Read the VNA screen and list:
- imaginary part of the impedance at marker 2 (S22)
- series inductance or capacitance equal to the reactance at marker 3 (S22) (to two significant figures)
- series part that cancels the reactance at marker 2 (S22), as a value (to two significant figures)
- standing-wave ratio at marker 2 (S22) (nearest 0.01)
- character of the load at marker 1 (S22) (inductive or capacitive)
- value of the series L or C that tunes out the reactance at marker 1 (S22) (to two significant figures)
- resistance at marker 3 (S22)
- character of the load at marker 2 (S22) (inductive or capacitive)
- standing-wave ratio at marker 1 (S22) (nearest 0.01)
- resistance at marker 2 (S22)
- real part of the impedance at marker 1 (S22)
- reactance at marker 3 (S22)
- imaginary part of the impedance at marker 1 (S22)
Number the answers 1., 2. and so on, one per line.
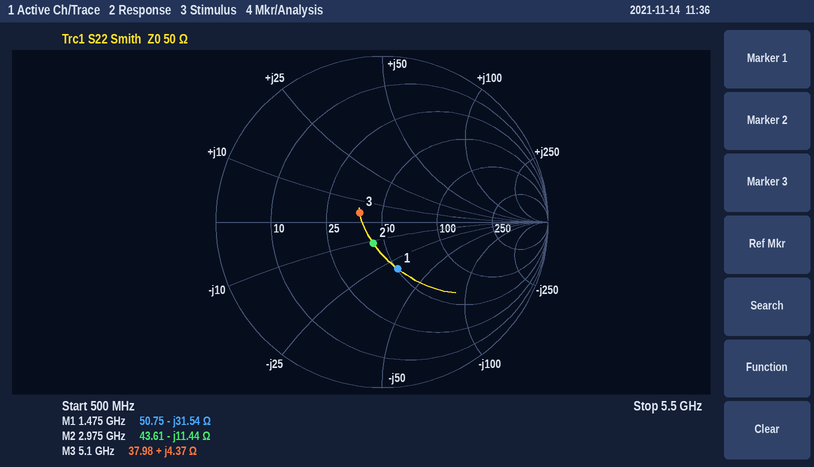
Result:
1. -11.44 Ω
2. 140 pH
3. 610 pH
4. 1.32
5. capacitive
6. 3.4 nH
7. 37.98 Ω
8. capacitive
9. 1.85
10. 43.61 Ω
11. 50.75 Ω
12. +4.37 Ω
13. -31.54 Ω
